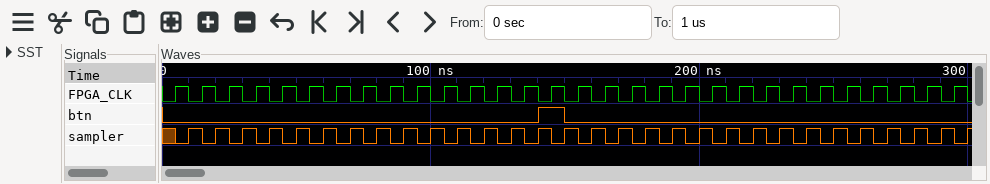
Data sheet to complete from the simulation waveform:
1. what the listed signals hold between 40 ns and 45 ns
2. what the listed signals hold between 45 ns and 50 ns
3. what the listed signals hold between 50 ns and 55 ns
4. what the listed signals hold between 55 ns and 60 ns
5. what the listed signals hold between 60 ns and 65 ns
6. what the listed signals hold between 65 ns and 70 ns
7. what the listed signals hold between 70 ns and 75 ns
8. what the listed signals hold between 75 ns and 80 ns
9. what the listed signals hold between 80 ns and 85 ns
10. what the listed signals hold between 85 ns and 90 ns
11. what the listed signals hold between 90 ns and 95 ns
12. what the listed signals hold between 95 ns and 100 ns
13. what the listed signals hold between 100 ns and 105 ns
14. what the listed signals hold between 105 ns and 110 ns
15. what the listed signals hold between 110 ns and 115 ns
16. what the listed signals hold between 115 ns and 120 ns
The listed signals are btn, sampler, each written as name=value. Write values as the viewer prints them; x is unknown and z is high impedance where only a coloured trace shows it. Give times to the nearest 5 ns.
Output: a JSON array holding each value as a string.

["btn=0, sampler=1", "btn=0, sampler=0", "btn=0, sampler=1", "btn=0, sampler=0", "btn=0, sampler=1", "btn=0, sampler=0", "btn=0, sampler=1", "btn=0, sampler=0", "btn=0, sampler=1", "btn=0, sampler=0", "btn=0, sampler=1", "btn=0, sampler=0", "btn=0, sampler=1", "btn=0, sampler=0", "btn=0, sampler=1", "btn=0, sampler=0"]
